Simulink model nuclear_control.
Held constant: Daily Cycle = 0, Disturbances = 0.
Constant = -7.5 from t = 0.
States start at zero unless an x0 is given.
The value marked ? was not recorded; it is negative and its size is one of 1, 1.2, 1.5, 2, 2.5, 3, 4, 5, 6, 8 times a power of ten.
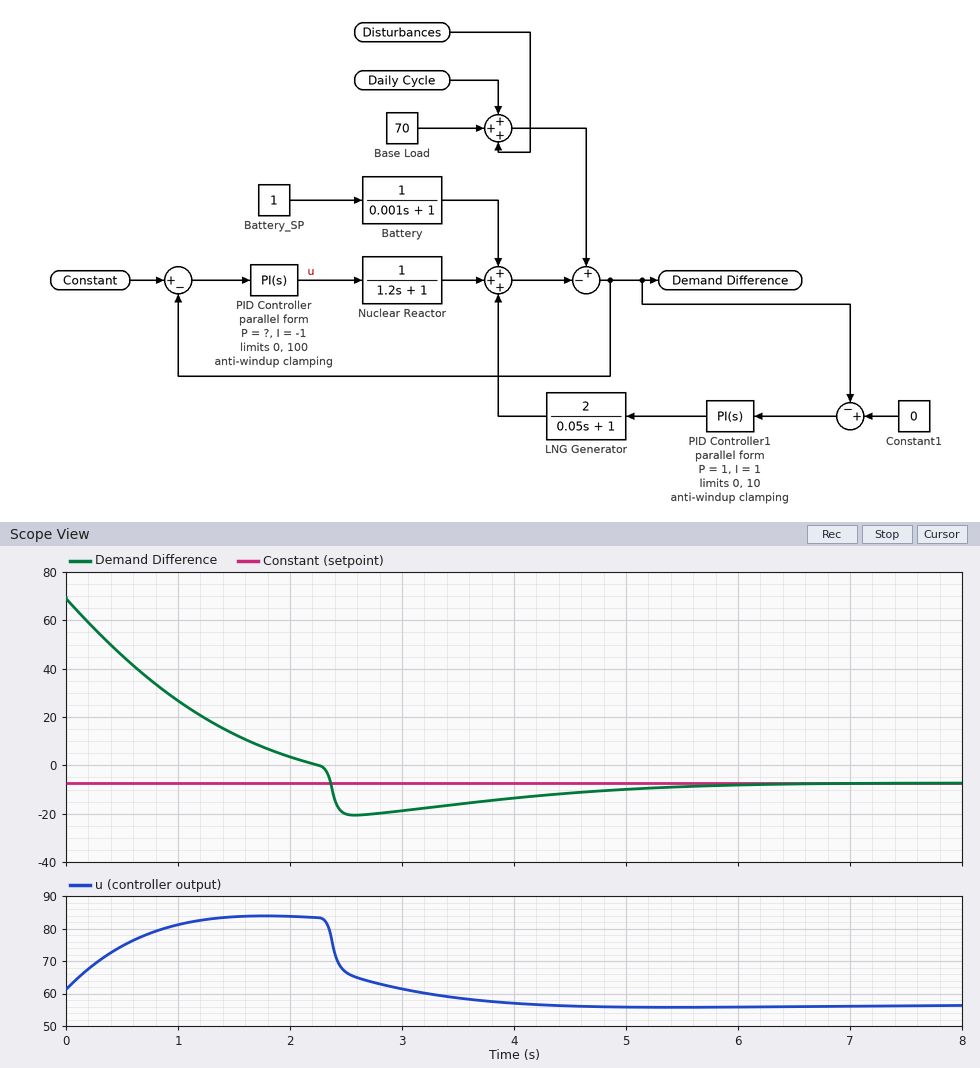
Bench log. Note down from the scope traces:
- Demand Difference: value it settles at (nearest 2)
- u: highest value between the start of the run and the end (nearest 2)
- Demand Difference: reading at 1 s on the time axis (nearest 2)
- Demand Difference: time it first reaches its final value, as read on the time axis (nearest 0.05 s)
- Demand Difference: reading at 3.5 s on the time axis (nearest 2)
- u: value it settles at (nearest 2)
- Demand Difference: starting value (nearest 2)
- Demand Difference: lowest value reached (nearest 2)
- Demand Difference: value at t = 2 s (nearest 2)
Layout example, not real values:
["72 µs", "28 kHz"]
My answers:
["-8", "84", "26", "2.35 s", "-16", "56", "70", "-20", "4"]
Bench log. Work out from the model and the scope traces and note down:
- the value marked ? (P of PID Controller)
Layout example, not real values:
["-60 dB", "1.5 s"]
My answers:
["-0.8"]
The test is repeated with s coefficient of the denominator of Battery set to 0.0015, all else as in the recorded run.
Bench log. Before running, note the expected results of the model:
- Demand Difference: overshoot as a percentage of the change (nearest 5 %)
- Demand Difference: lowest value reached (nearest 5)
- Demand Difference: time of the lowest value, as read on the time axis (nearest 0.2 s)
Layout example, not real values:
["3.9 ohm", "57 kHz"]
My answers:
["15 %", "-20", "2.6 s"]
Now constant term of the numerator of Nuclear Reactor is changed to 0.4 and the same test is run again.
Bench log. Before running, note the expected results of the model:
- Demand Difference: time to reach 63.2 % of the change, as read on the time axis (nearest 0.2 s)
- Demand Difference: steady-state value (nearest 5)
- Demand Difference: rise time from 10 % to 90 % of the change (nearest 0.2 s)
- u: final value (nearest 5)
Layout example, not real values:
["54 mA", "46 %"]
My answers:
["1.4 s", "30", "2.8 s", "100"]
